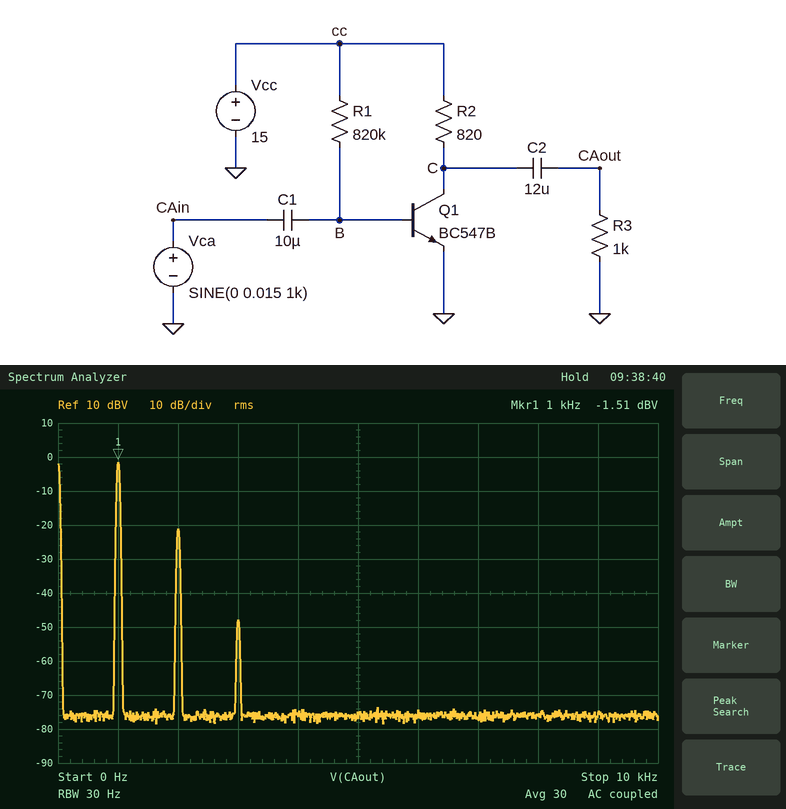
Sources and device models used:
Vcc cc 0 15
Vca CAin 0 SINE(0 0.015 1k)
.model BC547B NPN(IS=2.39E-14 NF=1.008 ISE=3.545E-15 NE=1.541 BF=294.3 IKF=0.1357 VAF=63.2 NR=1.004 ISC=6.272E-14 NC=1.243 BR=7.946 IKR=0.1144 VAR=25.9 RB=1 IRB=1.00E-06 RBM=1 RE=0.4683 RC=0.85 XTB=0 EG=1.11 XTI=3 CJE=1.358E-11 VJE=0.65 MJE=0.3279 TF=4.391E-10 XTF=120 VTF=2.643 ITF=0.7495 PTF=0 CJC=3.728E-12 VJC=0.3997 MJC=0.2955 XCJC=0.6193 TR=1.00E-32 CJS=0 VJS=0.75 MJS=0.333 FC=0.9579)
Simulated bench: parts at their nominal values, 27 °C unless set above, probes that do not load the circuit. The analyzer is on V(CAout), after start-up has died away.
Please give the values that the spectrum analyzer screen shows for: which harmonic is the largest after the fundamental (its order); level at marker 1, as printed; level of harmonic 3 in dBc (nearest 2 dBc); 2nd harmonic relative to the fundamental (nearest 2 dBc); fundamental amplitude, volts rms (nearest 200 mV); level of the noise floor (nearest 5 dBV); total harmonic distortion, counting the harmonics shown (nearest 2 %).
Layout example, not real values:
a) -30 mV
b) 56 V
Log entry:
a) 2
b) -1.51 dBV
c) -46 dBc
d) -20 dBc
e) 800 mV
f) -75 dBV
g) 10 %
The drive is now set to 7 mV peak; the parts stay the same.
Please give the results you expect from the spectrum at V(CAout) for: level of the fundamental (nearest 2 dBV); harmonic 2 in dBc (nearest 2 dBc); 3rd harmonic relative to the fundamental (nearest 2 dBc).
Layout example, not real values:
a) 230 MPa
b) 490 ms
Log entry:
a) -8 dBV
b) -26 dBc
c) -60 dBc
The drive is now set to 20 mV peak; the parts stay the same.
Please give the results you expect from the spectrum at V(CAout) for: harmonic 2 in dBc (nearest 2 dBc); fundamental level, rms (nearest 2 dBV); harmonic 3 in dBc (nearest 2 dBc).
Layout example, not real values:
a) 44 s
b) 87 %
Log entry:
a) -18 dBc
b) 0 dBV
c) -42 dBc
